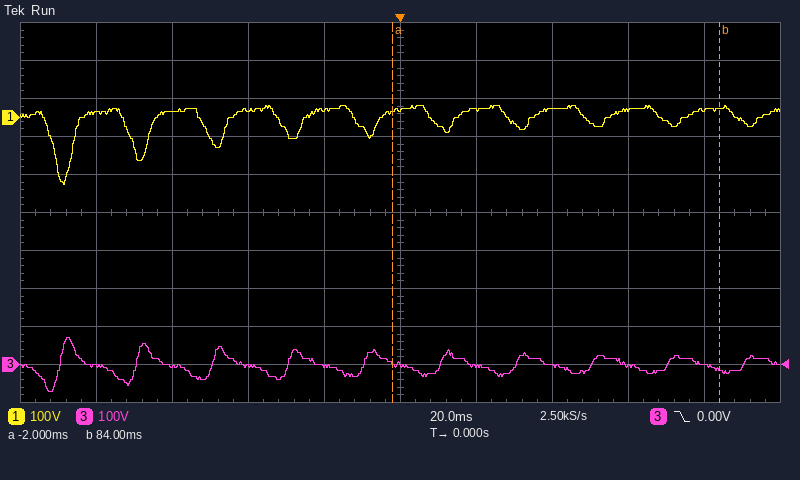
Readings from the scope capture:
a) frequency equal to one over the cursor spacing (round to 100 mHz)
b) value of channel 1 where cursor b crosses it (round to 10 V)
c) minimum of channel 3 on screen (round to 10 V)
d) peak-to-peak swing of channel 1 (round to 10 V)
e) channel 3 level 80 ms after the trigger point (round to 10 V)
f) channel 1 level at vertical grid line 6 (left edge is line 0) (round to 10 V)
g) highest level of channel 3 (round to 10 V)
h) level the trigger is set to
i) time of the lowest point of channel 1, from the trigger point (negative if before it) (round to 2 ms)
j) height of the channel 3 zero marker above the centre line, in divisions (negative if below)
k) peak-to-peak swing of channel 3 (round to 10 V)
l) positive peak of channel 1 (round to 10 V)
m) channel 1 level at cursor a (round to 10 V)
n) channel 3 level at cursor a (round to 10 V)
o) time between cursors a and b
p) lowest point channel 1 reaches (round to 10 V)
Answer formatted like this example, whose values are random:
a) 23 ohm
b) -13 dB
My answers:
a) 11.6 Hz
b) 20 V
c) -70 V
d) 210 V
e) 0 V
f) 20 V
g) 70 V
h) 0.00 V
i) -88 ms
j) -4.0 div
k) 140 V
l) 30 V
m) 20 V
n) 0 V
o) 86 ms
p) -180 V
